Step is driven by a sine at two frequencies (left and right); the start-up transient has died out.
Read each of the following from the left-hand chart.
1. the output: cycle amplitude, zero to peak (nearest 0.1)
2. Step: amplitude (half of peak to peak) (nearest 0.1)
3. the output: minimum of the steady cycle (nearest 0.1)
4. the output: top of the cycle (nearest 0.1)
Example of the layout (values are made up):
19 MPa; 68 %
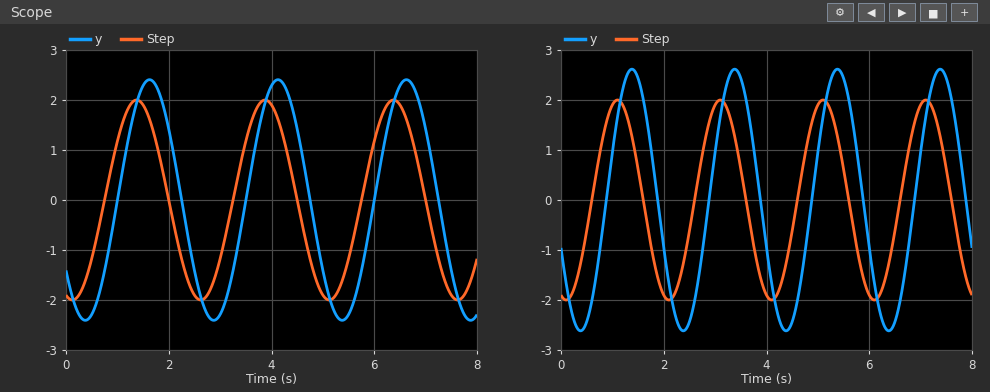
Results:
2.4; 2.0; -2.4; 2.4
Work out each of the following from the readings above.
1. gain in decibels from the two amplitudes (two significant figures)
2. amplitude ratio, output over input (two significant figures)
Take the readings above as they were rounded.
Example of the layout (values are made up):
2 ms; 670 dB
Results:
1.6 dB; 1.2
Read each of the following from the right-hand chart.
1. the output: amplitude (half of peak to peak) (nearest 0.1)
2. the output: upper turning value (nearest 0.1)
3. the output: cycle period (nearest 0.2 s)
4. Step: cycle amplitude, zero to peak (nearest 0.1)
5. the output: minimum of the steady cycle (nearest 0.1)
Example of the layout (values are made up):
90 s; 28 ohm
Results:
2.6; 2.6; 2.0 s; 2.0; -2.6
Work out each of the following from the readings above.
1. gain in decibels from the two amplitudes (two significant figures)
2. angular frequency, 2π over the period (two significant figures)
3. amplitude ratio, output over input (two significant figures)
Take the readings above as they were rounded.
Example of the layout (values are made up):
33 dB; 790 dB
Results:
2.3 dB; 3.1 rad/s; 1.3
